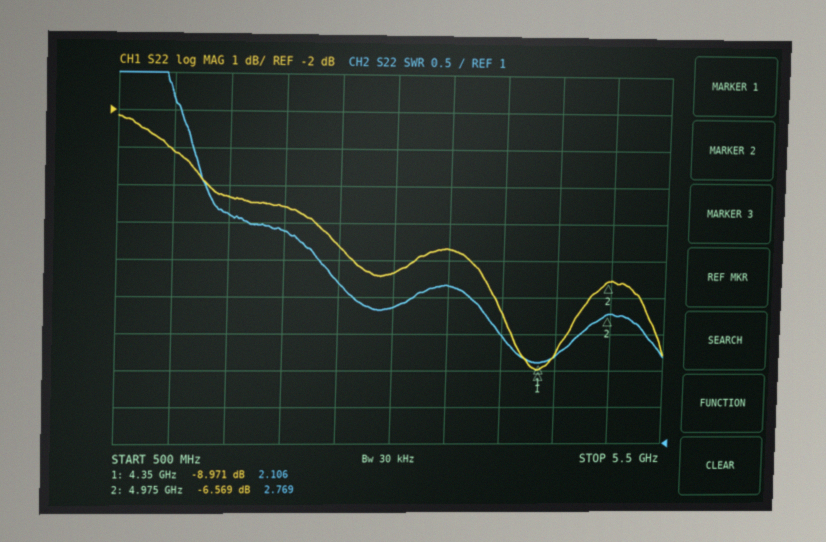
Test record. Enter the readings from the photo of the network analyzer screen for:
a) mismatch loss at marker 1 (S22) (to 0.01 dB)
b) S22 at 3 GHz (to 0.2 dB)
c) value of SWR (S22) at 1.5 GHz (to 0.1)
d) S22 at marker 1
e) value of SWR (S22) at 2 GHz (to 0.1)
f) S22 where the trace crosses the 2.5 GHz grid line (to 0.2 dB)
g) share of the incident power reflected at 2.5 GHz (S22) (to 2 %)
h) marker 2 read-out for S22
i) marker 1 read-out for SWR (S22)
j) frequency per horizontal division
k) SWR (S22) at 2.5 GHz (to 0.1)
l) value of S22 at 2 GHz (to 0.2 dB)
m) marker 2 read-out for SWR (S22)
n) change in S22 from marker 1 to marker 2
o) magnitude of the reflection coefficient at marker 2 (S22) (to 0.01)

0.59 dB
-6.4 dB
4.1
-8.971 dB
3.9
-5.6 dB
28 %
-6.569 dB
2.106
500 MHz
3.2
-4.6 dB
2.769
2.402 dB
0.47
